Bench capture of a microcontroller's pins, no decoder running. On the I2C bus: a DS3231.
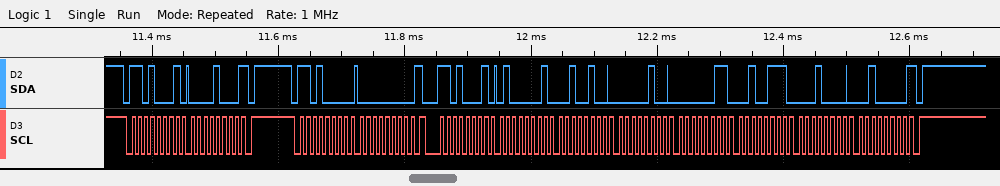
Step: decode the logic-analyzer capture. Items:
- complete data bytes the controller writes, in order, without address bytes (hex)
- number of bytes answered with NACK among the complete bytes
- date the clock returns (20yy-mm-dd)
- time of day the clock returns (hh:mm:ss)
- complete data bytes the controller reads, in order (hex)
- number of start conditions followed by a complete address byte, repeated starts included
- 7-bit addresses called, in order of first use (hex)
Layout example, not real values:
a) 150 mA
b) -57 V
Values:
a) 00
b) 2
c) 2020-10-27
d) 04:24:41
e) 08 41 24 04 03 27 10 20
f) 3
g) 0x68
